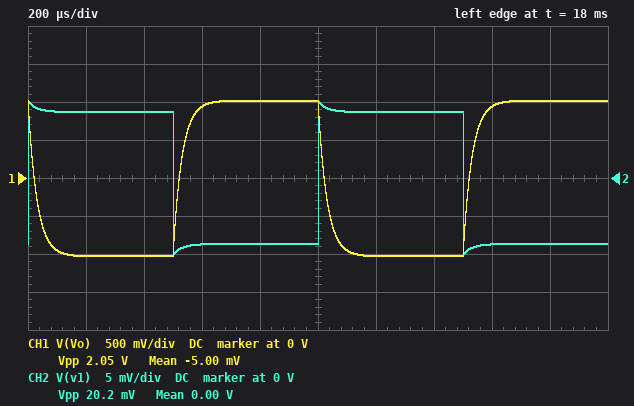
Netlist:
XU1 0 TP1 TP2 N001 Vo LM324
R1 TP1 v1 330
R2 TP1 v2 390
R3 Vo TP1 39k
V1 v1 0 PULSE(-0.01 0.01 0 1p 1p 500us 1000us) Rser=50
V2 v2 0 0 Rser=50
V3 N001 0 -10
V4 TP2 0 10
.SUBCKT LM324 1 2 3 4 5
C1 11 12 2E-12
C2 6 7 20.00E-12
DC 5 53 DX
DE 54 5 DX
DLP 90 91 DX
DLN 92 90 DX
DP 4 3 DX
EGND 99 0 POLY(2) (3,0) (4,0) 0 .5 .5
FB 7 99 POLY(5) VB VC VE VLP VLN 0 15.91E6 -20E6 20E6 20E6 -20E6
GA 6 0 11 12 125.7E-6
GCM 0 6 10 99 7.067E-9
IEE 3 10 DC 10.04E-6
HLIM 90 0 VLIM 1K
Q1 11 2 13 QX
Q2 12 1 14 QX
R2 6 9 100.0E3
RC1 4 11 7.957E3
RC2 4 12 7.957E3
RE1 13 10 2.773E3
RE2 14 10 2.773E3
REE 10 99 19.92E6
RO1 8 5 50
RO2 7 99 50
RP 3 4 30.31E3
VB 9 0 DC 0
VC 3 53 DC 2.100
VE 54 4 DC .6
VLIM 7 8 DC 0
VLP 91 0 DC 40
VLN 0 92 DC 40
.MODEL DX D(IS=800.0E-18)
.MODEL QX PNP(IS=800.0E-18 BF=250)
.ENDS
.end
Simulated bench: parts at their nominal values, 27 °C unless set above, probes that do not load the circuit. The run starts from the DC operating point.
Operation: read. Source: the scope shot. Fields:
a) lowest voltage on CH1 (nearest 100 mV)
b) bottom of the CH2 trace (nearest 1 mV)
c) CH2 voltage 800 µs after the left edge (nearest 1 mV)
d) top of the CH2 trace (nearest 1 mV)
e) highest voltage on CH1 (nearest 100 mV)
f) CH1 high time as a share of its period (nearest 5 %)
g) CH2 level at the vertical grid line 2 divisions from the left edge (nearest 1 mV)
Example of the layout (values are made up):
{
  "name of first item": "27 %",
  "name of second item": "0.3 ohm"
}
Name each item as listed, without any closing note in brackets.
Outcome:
{
  "lowest voltage on CH1": "-1.0 V",
  "bottom of the CH2 trace": "-10 mV",
  "CH2 voltage 800 µs after the left edge": "-9 mV",
  "top of the CH2 trace": "10 mV",
  "highest voltage on CH1": "1.0 V",
  "CH1 high time as a share of its period": "50 %",
  "CH2 level at the vertical grid line 2 divisions from the left edge": "9 mV"
}
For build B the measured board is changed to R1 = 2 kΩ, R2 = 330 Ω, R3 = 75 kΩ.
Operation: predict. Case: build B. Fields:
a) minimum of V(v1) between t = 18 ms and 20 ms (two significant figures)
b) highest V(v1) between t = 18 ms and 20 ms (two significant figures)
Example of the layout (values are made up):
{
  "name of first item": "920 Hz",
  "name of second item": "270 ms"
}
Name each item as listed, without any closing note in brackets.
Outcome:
{
  "minimum of V(v1) between t = 18 ms and 20 ms": "-9.8 mV",
  "highest V(v1) between t = 18 ms and 20 ms": "9.8 mV"
}
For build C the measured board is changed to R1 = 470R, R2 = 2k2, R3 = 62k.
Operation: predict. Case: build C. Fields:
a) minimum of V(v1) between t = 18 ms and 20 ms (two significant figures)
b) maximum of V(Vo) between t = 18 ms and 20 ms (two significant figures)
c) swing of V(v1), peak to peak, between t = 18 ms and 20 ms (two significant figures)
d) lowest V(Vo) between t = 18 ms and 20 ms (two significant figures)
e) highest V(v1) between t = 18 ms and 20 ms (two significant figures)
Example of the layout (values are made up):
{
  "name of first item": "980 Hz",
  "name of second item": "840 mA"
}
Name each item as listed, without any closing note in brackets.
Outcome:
{
  "minimum of V(v1) between t = 18 ms and 20 ms": "-11 mV",
  "maximum of V(Vo) between t = 18 ms and 20 ms": "1.2 V",
  "swing of V(v1), peak to peak, between t = 18 ms and 20 ms": "21 mV",
  "lowest V(Vo) between t = 18 ms and 20 ms": "-1.2 V",
  "highest V(v1) between t = 18 ms and 20 ms": "11 mV"
}
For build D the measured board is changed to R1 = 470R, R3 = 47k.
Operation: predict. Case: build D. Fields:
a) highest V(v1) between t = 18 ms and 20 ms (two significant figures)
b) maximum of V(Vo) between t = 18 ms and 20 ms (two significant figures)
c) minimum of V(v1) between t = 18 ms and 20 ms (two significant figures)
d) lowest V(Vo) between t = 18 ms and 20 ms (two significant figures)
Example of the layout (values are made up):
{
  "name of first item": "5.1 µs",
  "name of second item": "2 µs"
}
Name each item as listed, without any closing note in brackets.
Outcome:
{
  "highest V(v1) between t = 18 ms and 20 ms": "9.9 mV",
  "maximum of V(Vo) between t = 18 ms and 20 ms": "890 mV",
  "minimum of V(v1) between t = 18 ms and 20 ms": "-9.9 mV",
  "lowest V(Vo) between t = 18 ms and 20 ms": "-910 mV"
}
